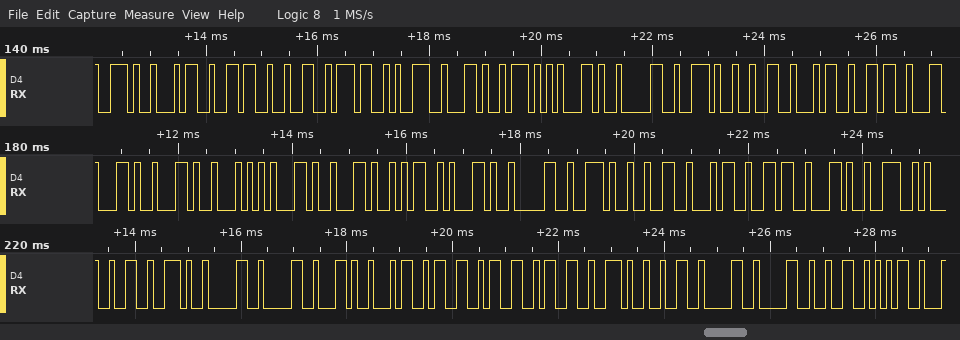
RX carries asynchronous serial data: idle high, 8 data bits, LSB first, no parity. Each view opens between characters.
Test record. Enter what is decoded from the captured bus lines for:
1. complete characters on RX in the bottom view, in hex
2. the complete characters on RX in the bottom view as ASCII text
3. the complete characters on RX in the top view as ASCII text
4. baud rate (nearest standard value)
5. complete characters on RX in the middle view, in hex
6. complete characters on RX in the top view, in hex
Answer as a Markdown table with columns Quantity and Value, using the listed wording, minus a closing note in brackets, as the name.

| Quantity | Value |
|---|---|
| complete characters on RX in the bottom view, in hex | 32, 2E, 30, 30, 2C, 34, 33, 33, 33, 2E, 32, 30, 30, 32, 35 |
| the complete characters on RX in the bottom view as ASCII text | "2.00,4333.20025" |
| the complete characters on RX in the top view as ASCII text | ".46279,W,0.246" |
| baud rate | 9600 baud |
| complete characters on RX in the middle view, in hex | 2C, 2C, 54, 2C, 2C, 4D, 2C, 30, 2E, 32, 34, 36, 2C, 4E |
| complete characters on RX in the top view, in hex | 2E, 34, 36, 32, 37, 39, 2C, 57, 2C, 30, 2E, 32, 34, 36 |
